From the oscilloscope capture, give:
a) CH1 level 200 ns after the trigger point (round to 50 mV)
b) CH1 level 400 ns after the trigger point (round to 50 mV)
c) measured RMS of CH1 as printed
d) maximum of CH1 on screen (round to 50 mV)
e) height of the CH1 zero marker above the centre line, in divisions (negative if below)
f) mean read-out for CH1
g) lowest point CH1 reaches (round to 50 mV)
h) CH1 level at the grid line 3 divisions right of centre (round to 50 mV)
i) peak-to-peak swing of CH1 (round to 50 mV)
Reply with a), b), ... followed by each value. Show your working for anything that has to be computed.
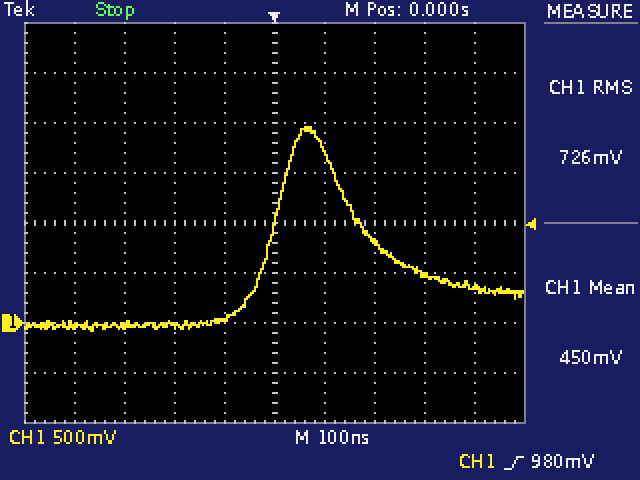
a) 800 mV
b) 350 mV
c) 726 mV
d) 1.95 V
e) -2.0 div
f) 450 mV
g) -100 mV
h) 500 mV
i) 1.95 V − (-100 mV) = 2.05 V
